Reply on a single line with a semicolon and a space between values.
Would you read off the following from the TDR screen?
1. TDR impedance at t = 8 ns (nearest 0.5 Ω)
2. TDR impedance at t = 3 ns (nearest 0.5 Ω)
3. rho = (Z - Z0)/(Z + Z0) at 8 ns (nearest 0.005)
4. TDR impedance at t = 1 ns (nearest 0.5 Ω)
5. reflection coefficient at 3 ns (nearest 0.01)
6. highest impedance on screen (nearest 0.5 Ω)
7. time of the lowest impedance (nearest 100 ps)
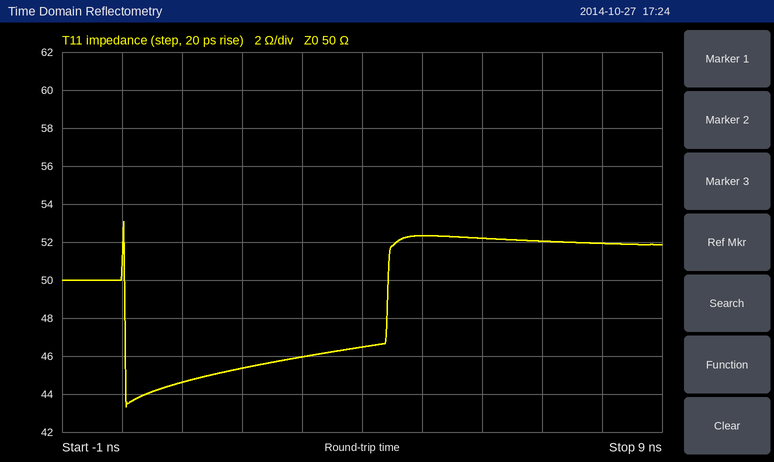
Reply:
52.0 Ω; 46.0 Ω; +0.020; 44.5 Ω; -0.04; 53.0 Ω; 100 ps
